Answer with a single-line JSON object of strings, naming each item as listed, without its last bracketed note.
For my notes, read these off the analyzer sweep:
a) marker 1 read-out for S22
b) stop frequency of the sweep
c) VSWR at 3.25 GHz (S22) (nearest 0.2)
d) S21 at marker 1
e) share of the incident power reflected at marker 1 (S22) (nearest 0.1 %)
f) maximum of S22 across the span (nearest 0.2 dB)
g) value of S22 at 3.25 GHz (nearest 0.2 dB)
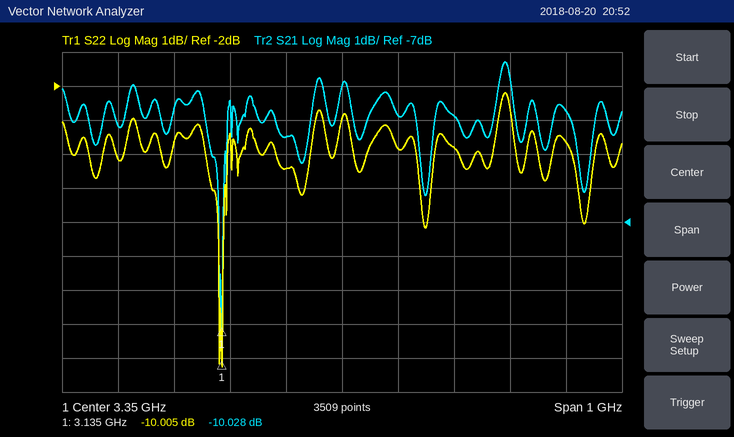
{"marker 1 read-out for S22": "-10.005 dB", "stop frequency of the sweep": "3.85 GHz", "VSWR at 3.25 GHz (S22)": "4.0", "S21 at marker 1": "-10.028 dB", "share of the incident power reflected at marker 1 (S22)": "10.0 %", "maximum of S22 across the span": "-2.2 dB", "value of S22 at 3.25 GHz": "-4.4 dB"}
